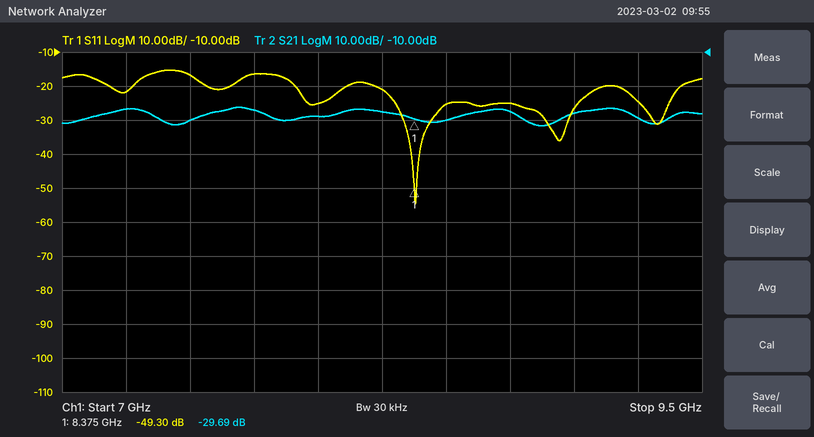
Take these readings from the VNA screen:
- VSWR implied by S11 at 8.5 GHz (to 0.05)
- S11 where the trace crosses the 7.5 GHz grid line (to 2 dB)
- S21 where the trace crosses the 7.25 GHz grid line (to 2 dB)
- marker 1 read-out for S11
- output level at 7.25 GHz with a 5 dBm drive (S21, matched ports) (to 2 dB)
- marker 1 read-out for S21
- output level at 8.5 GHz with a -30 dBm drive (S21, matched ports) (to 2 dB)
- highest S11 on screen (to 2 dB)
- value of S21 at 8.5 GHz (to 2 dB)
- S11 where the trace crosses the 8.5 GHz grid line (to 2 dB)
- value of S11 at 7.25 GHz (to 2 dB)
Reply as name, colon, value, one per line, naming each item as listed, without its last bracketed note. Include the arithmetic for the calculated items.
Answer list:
VSWR implied by S11 at 8.5 GHz: |Γ| = 10^(-26/20) = 0.0501; VSWR = (1 + 0.0501)/(1 − 0.0501) ≈ 1.11, so 1.10 to the nearest 0.05
S11 where the trace crosses the 7.5 GHz grid line: -16 dB
S21 where the trace crosses the 7.25 GHz grid line: -26 dB
marker 1 read-out for S11: -49.30 dB
output level at 7.25 GHz with a 5 dBm drive (S21, matched ports): 5 dBm + (-26 dB) = -22 dBm
marker 1 read-out for S21: -29.69 dB
output level at 8.5 GHz with a -30 dBm drive (S21, matched ports): -30 dBm + (-30 dB) = -60 dBm
highest S11 on screen: -16 dB
value of S21 at 8.5 GHz: -30 dB
S11 where the trace crosses the 8.5 GHz grid line: -26 dB
value of S11 at 7.25 GHz: -22 dB
